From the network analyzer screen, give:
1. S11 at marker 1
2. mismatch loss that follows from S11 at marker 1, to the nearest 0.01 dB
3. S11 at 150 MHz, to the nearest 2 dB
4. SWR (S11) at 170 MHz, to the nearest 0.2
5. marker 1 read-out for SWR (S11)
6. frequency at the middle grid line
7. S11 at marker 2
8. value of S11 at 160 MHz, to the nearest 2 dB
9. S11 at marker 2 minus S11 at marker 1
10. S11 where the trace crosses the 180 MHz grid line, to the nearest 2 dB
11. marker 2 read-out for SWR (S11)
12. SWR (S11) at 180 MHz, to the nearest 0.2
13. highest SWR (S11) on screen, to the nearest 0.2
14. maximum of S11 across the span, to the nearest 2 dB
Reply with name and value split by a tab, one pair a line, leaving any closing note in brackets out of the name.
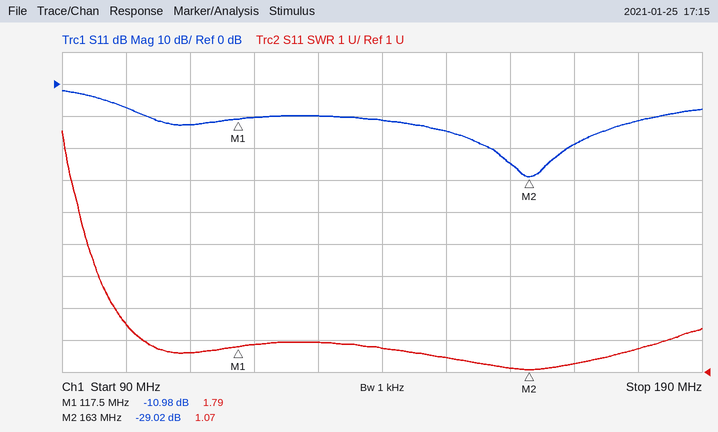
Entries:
S11 at marker 1	-10.98 dB
mismatch loss that follows from S11 at marker 1, to the nearest 0.01 dB	0.36 dB
S11 at 150 MHz, to the nearest 2 dB	-14 dB
SWR (S11) at 170 MHz, to the nearest 0.2	1.2
marker 1 read-out for SWR	1.79
frequency at the middle grid line	140 MHz
S11 at marker 2	-29.02 dB
value of S11 at 160 MHz, to the nearest 2 dB	-24 dB
S11 at marker 2 minus S11 at marker 1	-18.04 dB
S11 where the trace crosses the 180 MHz grid line, to the nearest 2 dB	-12 dB
marker 2 read-out for SWR	1.07
SWR (S11) at 180 MHz, to the nearest 0.2	1.8
highest SWR (S11) on screen, to the nearest 0.2	8.6
maximum of S11 across the span, to the nearest 2 dB	-2 dB
